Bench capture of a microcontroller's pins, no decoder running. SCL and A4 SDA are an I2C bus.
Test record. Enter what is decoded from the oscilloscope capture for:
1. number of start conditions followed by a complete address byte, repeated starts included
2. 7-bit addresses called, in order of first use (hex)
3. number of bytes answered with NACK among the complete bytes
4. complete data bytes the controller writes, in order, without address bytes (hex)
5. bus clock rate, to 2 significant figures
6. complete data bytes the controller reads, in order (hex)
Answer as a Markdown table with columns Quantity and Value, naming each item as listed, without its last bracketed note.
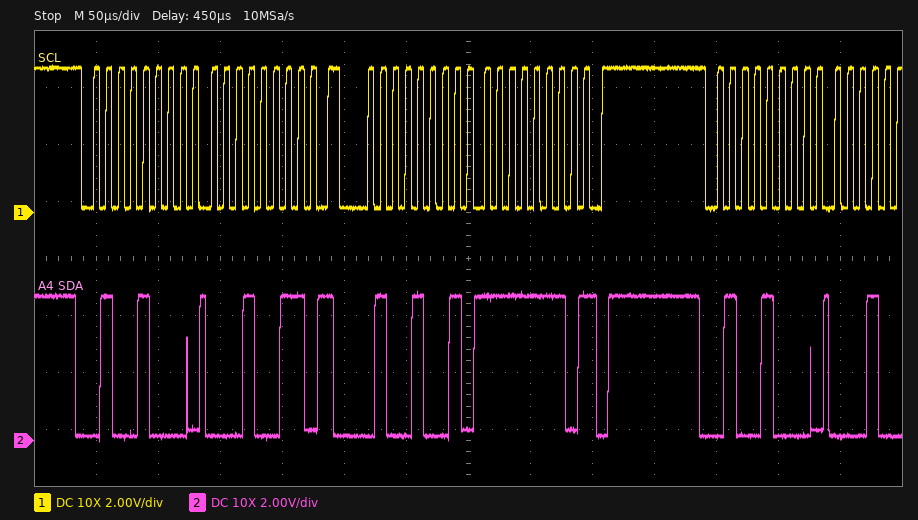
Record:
| Quantity | Value |
|---|---|
| number of start conditions followed by a complete address byte, repeated starts included | 3 |
| 7-bit addresses called, in order of first use | 0x24 |
| number of bytes answered with NACK among the complete bytes | 1 |
| complete data bytes the controller writes, in order, without address bytes | 13 |
| bus clock rate, to 2 significant figures | 100 kHz |
| complete data bytes the controller reads, in order | FE |
